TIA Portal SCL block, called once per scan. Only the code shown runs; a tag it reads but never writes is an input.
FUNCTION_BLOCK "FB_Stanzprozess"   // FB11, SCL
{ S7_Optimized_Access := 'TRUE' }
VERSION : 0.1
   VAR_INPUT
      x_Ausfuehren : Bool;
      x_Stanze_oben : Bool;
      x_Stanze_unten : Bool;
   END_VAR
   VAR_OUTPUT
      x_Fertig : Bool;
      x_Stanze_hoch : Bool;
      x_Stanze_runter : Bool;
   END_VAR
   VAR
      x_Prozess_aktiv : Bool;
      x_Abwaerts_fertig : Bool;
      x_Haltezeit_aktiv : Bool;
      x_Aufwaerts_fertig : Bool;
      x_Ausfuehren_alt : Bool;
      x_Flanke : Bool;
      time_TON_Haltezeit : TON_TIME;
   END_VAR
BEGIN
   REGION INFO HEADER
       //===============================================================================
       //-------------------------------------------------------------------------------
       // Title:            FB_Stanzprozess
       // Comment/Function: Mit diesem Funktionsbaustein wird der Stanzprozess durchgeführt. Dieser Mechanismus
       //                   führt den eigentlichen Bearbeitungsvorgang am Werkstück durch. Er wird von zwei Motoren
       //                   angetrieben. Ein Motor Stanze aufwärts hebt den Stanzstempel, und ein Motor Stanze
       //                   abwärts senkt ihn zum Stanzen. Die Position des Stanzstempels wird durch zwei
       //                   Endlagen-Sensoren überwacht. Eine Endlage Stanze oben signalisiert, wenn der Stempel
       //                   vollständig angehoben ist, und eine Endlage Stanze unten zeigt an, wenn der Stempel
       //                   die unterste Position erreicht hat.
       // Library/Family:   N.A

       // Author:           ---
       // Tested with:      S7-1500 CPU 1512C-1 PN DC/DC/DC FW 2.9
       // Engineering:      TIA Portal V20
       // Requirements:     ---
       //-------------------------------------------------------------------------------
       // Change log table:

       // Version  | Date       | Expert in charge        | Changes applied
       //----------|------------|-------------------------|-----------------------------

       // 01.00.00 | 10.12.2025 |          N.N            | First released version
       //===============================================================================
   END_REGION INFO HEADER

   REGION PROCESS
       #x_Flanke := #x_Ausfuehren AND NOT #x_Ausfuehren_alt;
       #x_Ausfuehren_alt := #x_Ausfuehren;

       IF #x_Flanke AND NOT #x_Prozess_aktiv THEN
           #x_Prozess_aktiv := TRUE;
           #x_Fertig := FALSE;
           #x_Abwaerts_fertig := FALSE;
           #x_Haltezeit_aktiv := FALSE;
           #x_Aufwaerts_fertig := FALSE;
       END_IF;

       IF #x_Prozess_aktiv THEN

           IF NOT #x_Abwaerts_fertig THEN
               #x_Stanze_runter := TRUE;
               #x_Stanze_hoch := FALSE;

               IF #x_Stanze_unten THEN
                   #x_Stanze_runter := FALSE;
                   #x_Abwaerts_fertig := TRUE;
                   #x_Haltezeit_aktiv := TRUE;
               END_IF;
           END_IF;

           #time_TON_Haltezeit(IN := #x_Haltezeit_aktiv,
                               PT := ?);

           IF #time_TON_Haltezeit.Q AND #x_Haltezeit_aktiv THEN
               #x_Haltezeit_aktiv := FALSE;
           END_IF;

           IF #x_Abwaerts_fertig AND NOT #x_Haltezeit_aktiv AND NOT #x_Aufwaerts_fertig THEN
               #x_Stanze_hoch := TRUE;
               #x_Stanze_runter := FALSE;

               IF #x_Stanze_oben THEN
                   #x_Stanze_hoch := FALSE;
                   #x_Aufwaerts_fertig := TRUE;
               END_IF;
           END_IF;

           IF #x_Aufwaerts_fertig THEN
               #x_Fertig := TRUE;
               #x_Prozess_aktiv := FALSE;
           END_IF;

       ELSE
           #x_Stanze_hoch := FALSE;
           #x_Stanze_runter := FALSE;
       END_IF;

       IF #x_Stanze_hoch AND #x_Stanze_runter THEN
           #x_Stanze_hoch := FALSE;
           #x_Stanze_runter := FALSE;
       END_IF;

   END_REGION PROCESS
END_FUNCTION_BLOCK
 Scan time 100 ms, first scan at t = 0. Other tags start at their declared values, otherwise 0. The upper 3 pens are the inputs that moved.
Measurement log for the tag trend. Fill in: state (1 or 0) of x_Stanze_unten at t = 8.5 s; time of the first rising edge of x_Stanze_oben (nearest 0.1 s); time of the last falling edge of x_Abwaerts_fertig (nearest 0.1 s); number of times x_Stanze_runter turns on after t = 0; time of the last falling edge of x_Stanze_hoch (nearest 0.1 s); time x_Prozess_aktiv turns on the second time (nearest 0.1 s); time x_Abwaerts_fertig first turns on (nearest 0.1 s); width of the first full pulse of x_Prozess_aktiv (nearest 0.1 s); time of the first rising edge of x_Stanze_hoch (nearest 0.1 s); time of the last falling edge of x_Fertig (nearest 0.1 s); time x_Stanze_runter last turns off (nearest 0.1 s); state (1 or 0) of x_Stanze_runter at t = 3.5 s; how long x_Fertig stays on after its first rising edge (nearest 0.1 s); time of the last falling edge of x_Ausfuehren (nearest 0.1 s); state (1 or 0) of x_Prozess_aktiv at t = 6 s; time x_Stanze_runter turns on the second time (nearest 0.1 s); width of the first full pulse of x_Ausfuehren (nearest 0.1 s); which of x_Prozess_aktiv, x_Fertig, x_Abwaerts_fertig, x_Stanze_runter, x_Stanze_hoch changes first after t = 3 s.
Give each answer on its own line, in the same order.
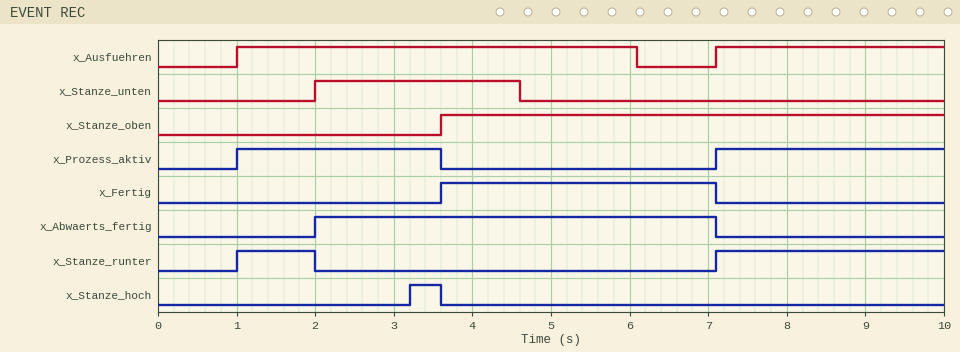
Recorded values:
0
3.6 s
7.1 s
2
3.6 s
7.1 s
2.0 s
2.6 s
3.2 s
7.1 s
2.0 s
0
3.5 s
6.1 s
0
7.1 s
5.1 s
x_Stanze_hoch
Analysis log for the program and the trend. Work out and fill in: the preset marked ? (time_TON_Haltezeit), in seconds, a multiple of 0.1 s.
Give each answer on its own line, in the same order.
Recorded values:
1.2 s
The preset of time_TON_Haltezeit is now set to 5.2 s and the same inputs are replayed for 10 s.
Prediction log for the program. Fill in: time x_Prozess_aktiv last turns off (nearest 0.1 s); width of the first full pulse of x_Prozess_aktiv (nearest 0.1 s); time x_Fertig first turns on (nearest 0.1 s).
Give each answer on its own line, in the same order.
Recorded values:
7.2 s
6.2 s
7.2 s
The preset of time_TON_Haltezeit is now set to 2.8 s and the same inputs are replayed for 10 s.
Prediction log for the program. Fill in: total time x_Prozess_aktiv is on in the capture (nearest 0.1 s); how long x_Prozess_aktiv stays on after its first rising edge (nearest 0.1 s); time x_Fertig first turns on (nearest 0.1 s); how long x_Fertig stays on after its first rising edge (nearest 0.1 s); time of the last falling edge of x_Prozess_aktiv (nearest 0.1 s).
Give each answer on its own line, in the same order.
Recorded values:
6.7 s
3.8 s
4.8 s
2.3 s
4.8 s
